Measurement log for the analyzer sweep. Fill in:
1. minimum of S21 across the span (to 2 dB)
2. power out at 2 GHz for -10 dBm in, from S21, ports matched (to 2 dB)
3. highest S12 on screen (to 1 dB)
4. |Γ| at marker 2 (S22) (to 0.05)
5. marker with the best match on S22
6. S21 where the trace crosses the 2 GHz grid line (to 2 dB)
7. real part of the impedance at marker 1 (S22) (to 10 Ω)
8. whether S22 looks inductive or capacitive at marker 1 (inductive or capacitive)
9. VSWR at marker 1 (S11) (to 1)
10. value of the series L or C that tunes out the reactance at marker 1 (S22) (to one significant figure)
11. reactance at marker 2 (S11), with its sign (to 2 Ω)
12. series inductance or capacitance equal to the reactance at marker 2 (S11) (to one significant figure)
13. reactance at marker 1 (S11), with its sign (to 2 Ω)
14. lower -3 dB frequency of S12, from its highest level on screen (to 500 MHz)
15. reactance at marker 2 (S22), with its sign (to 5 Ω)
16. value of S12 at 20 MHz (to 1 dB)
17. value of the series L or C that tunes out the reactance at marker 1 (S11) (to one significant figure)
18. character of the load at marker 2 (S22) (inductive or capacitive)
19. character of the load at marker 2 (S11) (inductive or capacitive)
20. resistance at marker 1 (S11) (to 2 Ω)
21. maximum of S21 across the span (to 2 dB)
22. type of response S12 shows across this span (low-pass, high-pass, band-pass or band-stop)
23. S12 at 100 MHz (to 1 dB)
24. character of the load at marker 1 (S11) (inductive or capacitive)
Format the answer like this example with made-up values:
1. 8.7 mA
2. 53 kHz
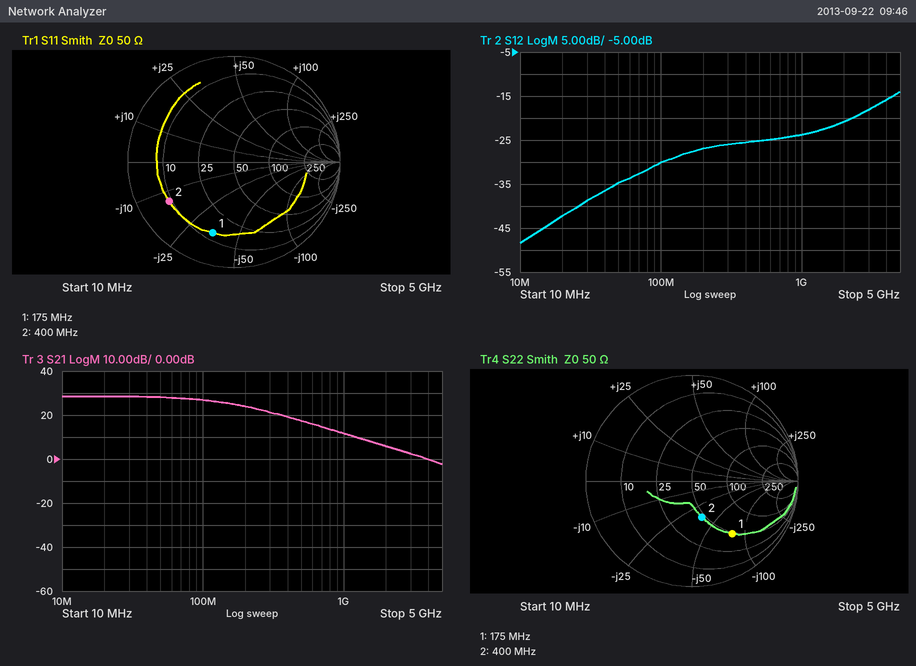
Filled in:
1. -2 dB
2. -4 dBm
3. -14 dB
4. 0.35
5. marker 2
6. 6 dB
7. 50 Ω
8. capacitive
9. 6
10. 70 nH
11. -14 Ω
12. 30 pF
13. -36 Ω
14. 3.5 GHz
15. -35 Ω
16. -42 dB
17. 30 nH
18. capacitive
19. capacitive
20. 14 Ω
21. 28 dB
22. high-pass
23. -30 dB
24. capacitive
